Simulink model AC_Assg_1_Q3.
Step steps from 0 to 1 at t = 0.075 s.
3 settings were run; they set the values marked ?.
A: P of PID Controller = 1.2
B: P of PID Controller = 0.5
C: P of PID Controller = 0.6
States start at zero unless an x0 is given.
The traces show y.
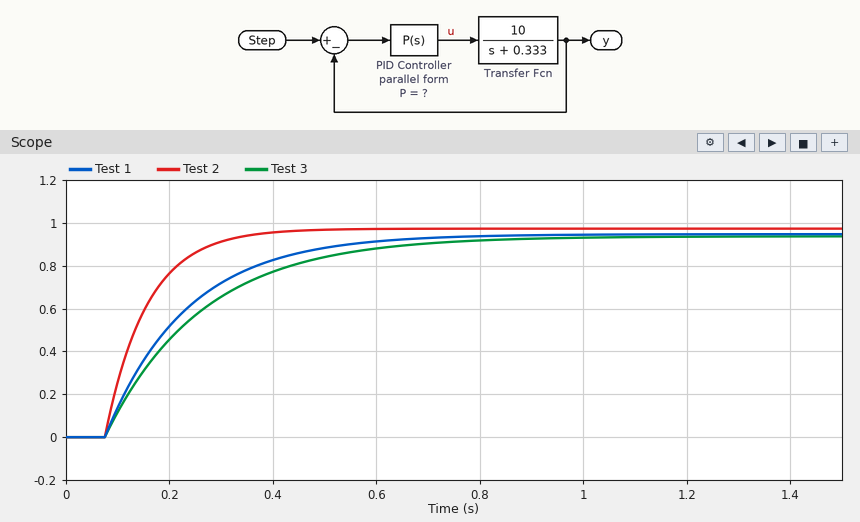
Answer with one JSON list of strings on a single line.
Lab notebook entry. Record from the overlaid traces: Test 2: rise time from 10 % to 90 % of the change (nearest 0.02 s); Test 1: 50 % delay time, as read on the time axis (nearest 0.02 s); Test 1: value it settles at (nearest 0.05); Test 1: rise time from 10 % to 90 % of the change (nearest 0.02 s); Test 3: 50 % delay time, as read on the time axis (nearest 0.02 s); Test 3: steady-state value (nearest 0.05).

["0.18 s", "0.18 s", "0.95", "0.34 s", "0.20 s", "0.95"]
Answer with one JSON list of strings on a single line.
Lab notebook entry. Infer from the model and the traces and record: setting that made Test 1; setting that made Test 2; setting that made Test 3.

["C", "A", "B"]
